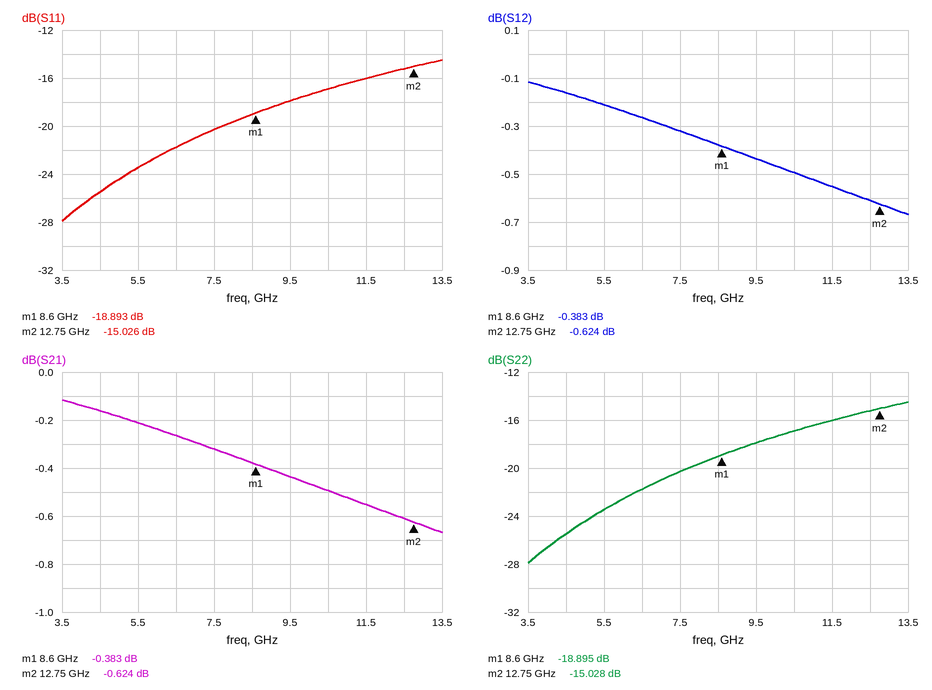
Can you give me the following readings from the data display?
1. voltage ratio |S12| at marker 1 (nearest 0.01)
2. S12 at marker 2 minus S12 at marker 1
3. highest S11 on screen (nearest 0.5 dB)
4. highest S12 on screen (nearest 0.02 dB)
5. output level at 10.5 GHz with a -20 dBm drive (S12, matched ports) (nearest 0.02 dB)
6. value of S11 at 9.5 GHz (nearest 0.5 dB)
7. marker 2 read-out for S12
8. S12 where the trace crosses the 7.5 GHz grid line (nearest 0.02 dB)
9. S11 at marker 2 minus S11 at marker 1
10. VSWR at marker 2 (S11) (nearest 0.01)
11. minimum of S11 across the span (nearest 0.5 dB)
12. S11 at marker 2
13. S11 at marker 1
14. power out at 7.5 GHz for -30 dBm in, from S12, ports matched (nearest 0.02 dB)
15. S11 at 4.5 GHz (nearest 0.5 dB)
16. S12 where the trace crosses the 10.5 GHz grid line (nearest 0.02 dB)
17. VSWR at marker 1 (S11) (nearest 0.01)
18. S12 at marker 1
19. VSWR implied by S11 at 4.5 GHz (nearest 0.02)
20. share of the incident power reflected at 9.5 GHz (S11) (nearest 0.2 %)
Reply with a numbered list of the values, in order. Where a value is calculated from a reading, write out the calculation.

1. 10^(-0.383/20) ≈ 0.96
2. -0.624 − (-0.383) = -0.241 dB
3. -14.5 dB
4. -0.12 dB
5. -20 dBm + (-0.50 dB) = -20.50 dBm
6. -18.0 dB
7. -0.624 dB
8. -0.32 dB
9. -15.026 − (-18.893) = 3.867 dB
10. (1 + 0.1773)/(1 − 0.1773) ≈ 1.43
11. -28.0 dB
12. -15.026 dB
13. -18.893 dB
14. -30 dBm + (-0.32 dB) = -30.32 dBm
15. -25.5 dB
16. -0.50 dB
17. (1 + 0.1136)/(1 − 0.1136) ≈ 1.26
18. -0.383 dB
19. |Γ| = 10^(-25.5/20) = 0.0531; VSWR = (1 + 0.0531)/(1 − 0.0531) ≈ 1.11, so 1.12 to the nearest 0.02
20. 10^(-18/10) ≈ 1.6 %
